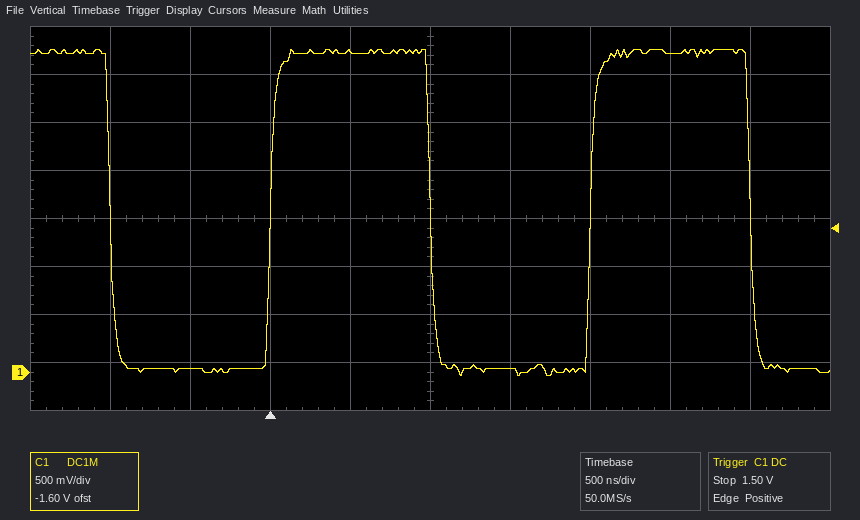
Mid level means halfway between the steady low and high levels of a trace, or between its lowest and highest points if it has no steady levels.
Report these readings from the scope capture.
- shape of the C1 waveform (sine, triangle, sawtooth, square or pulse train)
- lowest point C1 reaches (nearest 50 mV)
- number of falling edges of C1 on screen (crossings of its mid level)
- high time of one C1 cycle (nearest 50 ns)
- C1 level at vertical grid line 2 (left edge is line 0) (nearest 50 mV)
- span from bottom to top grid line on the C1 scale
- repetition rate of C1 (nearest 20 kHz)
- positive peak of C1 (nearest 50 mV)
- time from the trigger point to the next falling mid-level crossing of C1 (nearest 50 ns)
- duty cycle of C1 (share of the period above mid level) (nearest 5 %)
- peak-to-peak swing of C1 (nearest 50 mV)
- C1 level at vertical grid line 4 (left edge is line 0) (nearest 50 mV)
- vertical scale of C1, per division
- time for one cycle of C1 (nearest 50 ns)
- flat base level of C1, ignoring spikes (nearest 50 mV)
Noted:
square
-50 mV
3
1.00 µs
50 mV
4 V
500 kHz
3.35 V
1.00 µs
50 %
3.40 V
3.35 V
500 mV
2.00 µs
50 mV
